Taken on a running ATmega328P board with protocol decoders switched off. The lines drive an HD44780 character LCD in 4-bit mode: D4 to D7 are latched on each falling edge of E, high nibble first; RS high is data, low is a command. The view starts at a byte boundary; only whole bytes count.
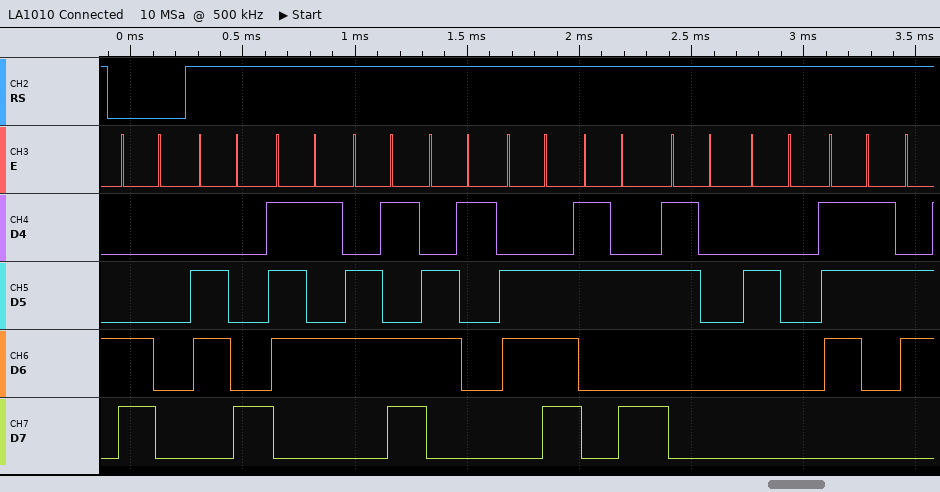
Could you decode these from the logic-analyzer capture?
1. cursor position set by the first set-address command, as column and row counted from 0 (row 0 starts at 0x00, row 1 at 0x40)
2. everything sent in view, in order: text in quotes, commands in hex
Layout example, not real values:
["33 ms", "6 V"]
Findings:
["column 0, row 1", "0xC0 \"human:0 s\""]
